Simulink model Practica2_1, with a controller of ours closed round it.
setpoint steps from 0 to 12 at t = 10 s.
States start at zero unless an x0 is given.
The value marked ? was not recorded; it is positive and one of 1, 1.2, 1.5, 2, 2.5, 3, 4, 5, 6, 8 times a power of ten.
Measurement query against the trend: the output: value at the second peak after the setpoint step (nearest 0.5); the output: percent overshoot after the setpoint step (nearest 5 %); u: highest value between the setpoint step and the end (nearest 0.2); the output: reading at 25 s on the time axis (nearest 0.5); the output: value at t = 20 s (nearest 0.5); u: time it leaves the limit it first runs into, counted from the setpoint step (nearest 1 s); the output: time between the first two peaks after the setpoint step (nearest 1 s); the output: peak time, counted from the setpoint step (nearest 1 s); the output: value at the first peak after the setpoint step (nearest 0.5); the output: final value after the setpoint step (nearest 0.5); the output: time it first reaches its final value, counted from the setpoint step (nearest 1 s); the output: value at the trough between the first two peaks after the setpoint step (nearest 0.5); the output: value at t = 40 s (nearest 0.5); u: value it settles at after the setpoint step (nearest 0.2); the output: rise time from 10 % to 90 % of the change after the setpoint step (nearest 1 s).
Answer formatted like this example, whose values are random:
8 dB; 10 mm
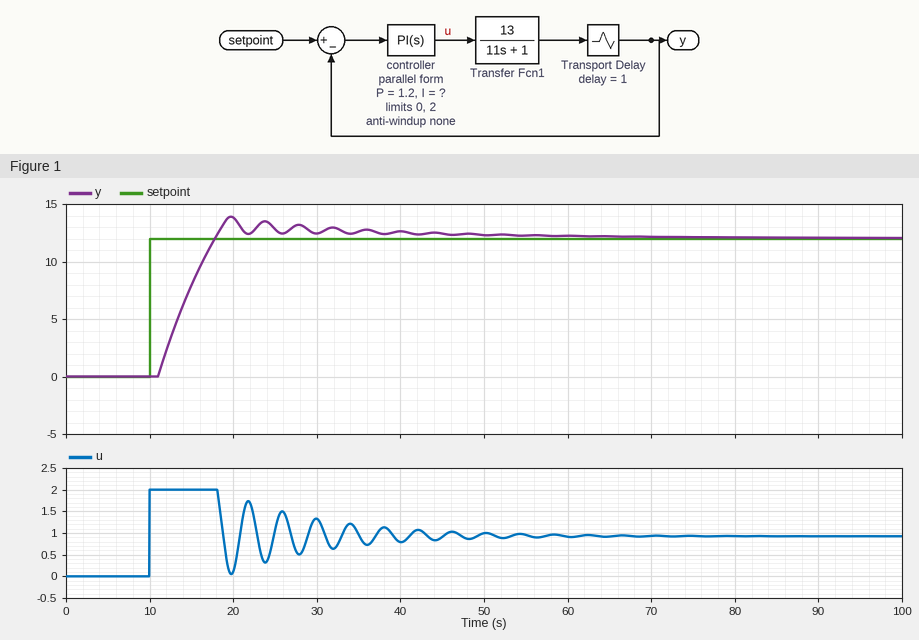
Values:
13.5; 15 %; 2.0; 13.0; 14.0; 8 s; 4 s; 10 s; 14.0; 12.0; 8 s; 12.5; 12.5; 1.0; 5 s
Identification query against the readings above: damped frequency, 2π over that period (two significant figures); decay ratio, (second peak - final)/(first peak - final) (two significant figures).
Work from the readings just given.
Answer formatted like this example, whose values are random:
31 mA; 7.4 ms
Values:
1.6 rad/s; 0.75
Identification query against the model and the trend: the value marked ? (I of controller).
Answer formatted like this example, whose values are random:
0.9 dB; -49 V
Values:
0.05
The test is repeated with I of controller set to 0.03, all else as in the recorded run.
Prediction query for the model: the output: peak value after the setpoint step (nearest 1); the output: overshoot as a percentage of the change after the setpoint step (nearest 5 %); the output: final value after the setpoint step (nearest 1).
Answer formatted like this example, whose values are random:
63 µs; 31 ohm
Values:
13; 10 %; 12
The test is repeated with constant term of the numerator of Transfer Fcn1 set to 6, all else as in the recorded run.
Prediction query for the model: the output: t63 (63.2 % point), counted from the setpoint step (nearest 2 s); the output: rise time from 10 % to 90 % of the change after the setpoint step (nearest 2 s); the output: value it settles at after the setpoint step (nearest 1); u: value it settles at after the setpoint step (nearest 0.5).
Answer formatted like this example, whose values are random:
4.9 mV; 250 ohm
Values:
12 s; 24 s; 12; 2.0
